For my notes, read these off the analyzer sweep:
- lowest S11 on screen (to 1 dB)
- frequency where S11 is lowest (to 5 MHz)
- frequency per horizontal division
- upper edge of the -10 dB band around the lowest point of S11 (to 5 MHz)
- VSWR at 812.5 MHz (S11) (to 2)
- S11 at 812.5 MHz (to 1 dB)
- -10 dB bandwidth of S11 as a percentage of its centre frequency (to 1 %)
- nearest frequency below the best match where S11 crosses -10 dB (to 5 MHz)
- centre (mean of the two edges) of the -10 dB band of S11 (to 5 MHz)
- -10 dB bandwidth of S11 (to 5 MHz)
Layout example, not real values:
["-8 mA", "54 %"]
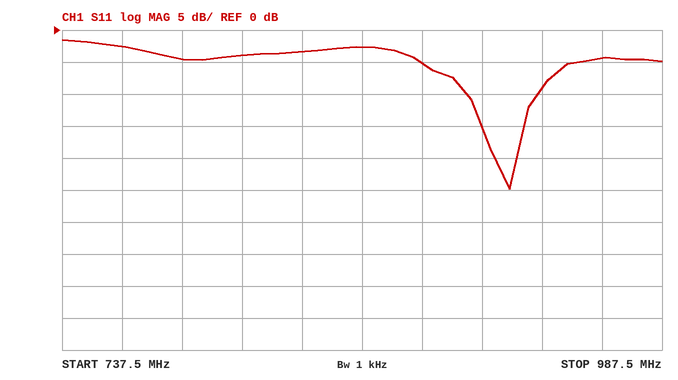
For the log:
["-25 dB", "925 MHz", "25 MHz", "935 MHz", "4", "-4 dB", "3 %", "905 MHz", "920 MHz", "30 MHz"]
